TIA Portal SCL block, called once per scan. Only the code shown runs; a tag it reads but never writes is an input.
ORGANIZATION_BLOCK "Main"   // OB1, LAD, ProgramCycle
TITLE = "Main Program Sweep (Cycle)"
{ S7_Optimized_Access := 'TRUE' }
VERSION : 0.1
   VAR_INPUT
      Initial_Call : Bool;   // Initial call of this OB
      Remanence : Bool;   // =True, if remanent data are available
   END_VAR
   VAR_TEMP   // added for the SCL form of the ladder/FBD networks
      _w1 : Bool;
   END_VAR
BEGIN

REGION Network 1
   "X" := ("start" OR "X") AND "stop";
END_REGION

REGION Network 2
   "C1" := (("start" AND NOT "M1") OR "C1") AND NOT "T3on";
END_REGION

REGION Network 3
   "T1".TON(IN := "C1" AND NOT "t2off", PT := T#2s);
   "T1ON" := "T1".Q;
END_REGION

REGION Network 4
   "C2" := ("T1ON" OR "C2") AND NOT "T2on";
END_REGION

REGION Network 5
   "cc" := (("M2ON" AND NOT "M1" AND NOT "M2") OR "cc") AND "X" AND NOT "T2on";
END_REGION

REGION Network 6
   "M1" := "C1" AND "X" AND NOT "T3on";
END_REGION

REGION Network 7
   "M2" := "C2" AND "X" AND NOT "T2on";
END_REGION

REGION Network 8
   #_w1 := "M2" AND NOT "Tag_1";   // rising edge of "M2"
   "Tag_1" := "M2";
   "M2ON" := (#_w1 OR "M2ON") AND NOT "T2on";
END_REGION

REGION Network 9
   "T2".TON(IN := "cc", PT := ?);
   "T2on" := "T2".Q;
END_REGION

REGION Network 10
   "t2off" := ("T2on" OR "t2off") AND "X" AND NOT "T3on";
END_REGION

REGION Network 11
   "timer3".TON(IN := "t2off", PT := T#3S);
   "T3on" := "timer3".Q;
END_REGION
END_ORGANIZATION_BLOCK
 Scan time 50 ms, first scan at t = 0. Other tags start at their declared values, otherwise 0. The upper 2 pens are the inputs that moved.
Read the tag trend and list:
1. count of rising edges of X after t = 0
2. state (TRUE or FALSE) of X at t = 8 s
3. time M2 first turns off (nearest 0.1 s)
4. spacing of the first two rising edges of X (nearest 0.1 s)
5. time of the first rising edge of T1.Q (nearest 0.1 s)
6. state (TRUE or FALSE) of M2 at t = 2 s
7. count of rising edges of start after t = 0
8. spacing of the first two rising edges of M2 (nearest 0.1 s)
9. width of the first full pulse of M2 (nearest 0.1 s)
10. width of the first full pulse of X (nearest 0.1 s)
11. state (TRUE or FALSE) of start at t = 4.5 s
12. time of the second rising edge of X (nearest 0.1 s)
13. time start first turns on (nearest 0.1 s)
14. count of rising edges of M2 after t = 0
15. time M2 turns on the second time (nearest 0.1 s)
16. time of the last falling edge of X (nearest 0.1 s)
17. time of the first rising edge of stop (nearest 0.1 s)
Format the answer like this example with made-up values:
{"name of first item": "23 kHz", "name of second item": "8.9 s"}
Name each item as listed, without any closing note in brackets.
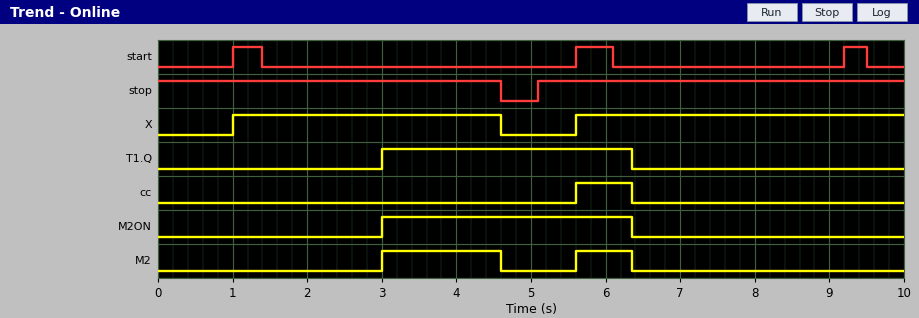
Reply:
{"count of rising edges of X after t = 0": "2", "state (TRUE or FALSE) of X at t = 8 s": "TRUE", "time M2 first turns off": "4.6 s", "spacing of the first two rising edges of X": "4.6 s", "time of the first rising edge of T1.Q": "3.0 s", "state (TRUE or FALSE) of M2 at t = 2 s": "FALSE", "count of rising edges of start after t = 0": "3", "spacing of the first two rising edges of M2": "2.6 s", "width of the first full pulse of M2": "1.6 s", "width of the first full pulse of X": "3.6 s", "state (TRUE or FALSE) of start at t = 4.5 s": "FALSE", "time of the second rising edge of X": "5.6 s", "time start first turns on": "1.0 s", "count of rising edges of M2 after t = 0": "2", "time M2 turns on the second time": "5.6 s", "time of the last falling edge of X": "4.6 s", "time of the first rising edge of stop": "5.1 s"}
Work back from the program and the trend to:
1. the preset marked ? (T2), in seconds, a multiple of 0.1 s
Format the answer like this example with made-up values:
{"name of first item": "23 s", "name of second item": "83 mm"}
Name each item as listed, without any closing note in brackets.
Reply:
{"the preset marked ? (T2), in seconds, a multiple of 0.1 s": "0.7 s"}
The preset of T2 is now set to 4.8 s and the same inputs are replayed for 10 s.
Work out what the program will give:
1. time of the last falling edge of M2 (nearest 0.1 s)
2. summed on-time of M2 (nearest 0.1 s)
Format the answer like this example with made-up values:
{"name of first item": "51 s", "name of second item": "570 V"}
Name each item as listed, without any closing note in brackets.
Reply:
{"time of the last falling edge of M2": "4.6 s", "summed on-time of M2": "6.0 s"}
